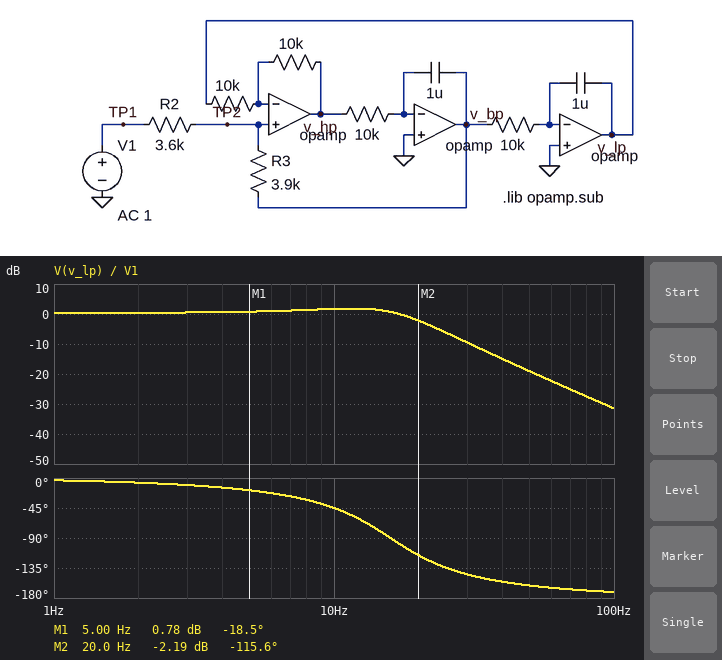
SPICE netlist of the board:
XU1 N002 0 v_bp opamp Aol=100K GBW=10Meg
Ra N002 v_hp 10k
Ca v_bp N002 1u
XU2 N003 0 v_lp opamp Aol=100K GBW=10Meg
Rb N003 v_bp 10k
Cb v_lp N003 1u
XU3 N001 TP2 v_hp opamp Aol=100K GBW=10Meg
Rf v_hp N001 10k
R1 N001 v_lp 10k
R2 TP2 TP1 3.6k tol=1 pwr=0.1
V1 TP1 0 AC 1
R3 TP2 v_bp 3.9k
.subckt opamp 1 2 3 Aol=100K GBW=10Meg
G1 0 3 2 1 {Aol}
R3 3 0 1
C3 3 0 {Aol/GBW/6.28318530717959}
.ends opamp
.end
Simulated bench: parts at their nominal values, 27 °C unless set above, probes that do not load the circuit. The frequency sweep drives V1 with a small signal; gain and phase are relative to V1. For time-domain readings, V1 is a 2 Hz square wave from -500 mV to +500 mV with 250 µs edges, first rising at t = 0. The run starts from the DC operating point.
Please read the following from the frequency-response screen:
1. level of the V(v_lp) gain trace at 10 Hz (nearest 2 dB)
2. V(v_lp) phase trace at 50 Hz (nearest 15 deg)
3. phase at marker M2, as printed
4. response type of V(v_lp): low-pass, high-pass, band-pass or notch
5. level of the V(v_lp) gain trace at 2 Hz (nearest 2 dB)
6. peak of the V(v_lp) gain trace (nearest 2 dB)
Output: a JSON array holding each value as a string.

["2 dB", "-165 deg", "-115.6 deg", "low-pass", "0 dB", "2 dB"]
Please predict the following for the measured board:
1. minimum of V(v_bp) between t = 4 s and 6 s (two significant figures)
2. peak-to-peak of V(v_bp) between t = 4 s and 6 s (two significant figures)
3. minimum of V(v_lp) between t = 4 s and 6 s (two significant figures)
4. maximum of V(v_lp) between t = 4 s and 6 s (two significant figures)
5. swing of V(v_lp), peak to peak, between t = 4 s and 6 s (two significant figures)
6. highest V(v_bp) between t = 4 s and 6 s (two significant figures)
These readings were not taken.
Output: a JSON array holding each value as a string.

["-580 mV", "1.2 V", "-710 mV", "710 mV", "1.4 V", "580 mV"]
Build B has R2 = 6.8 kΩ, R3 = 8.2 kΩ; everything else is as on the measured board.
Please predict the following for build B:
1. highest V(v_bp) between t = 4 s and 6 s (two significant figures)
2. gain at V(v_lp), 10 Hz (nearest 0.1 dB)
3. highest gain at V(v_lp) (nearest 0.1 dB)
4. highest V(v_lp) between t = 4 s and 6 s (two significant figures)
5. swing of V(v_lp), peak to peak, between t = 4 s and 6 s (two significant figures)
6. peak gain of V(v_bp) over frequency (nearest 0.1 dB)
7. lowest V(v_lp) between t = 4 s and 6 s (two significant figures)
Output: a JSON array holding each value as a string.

["630 mV", "2.4 dB", "2.6 dB", "770 mV", "1.5 V", "1.6 dB", "-770 mV"]
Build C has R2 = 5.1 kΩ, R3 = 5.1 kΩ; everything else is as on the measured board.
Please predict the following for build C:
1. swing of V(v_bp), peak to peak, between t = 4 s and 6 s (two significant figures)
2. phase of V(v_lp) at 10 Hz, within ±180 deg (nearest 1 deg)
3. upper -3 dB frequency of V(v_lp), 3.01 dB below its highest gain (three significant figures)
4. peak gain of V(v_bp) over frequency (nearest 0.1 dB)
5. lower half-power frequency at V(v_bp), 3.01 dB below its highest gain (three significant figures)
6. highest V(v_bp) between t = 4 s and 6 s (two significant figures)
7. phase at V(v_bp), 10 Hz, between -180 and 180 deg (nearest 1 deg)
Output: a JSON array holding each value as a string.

["1.1 V", "-46 deg", "18.6 Hz", "0 dB", "9.84 Hz", "550 mV", "-136 deg"]
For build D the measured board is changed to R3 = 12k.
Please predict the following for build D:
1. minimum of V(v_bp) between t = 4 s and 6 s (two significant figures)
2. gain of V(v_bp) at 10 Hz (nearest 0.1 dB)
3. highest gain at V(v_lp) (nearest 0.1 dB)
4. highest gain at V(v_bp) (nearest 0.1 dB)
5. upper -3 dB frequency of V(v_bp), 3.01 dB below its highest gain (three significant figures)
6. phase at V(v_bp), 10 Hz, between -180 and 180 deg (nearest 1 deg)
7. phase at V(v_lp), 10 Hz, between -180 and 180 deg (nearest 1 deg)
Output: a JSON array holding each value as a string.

["-1.1 V", "3.2 dB", "10.7 dB", "10.5 dB", "20.0 Hz", "-116 deg", "-26 deg"]
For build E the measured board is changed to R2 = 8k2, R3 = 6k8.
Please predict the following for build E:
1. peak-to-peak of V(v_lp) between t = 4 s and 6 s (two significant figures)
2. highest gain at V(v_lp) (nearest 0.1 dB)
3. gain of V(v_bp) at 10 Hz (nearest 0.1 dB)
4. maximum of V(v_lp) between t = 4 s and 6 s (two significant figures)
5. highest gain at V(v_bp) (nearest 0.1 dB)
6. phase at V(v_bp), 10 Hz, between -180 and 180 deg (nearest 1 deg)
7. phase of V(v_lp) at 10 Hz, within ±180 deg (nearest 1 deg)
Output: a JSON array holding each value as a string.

["1.1 V", "-0.1 dB", "-4.1 dB", "570 mV", "-1.6 dB", "-139 deg", "-49 deg"]
